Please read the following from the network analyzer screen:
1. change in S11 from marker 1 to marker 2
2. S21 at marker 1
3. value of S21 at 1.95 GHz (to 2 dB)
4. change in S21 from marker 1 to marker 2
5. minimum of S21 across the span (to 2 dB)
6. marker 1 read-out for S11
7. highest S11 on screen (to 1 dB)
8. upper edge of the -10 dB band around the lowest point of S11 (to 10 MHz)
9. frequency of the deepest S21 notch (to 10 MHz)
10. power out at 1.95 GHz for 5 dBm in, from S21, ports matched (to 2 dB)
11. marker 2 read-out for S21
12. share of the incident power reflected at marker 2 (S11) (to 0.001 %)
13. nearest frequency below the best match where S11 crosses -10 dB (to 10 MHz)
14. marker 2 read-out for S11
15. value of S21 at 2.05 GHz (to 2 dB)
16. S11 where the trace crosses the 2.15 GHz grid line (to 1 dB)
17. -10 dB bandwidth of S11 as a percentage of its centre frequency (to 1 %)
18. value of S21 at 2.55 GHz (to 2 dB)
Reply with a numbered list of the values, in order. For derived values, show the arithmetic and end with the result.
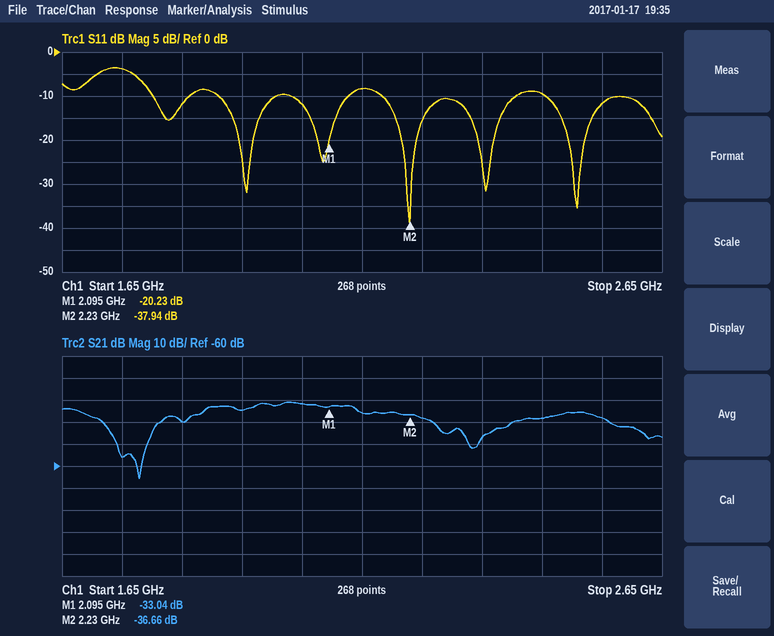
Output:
1. -37.94 − (-20.23) = -17.71 dB
2. -33.04 dB
3. -34 dB
4. -36.66 − (-33.04) = -3.62 dB
5. -66 dB
6. -20.23 dB
7. -4 dB
8. 2.41 GHz
9. 1.78 GHz
10. 5 dBm + (-34 dB) = -30 dBm
11. -36.66 dB
12. 10^(-37.94/10) ≈ 0.016 %
13. 2.18 GHz
14. -37.94 dB
15. -32 dB
16. -8 dB
17. 230 MHz / 2.295 GHz ≈ 10 %
18. -38 dB
